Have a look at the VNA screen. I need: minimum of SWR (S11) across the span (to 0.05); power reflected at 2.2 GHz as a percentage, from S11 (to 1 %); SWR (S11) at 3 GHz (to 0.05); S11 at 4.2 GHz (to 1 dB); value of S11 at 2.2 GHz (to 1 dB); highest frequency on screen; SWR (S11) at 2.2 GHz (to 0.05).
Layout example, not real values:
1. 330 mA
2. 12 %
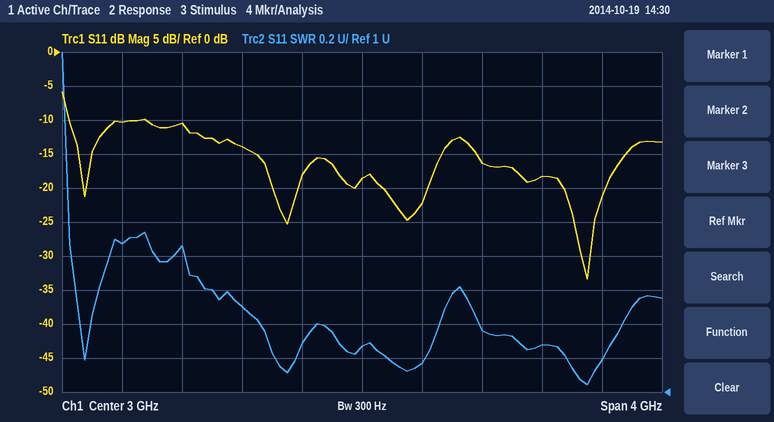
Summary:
1. 1.05
2. 4 %
3. 1.25
4. -18 dB
5. -14 dB
6. 5 GHz
7. 1.50
